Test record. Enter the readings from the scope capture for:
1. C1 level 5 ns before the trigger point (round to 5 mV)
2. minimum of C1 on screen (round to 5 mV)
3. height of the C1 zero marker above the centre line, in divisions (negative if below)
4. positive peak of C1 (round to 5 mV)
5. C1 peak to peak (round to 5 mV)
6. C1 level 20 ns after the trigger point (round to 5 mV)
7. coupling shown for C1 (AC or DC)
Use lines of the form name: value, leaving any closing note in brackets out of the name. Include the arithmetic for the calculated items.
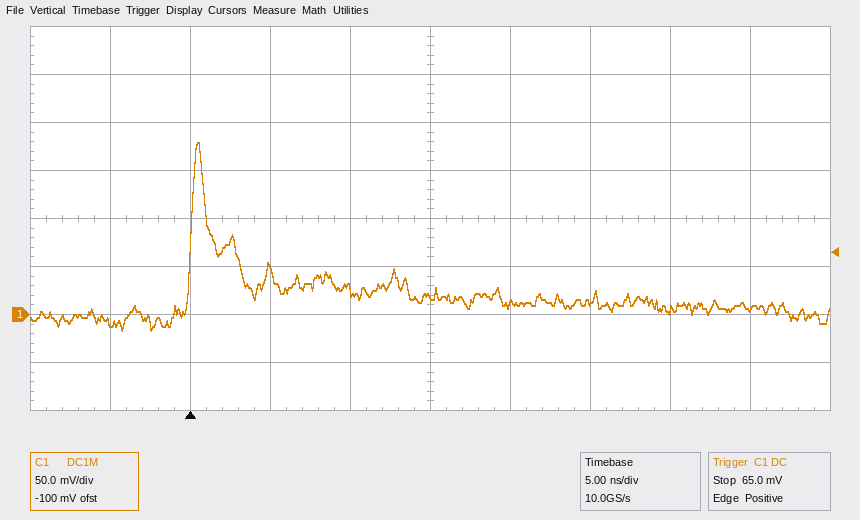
C1 level 5 ns before the trigger point: -10 mV
minimum of C1 on screen: -15 mV
height of the C1 zero marker above the centre line, in divisions: -2.0 div
positive peak of C1: 180 mV
C1 peak to peak: 180 mV − (-15 mV) = 195 mV
C1 level 20 ns after the trigger point: 10 mV
coupling shown for C1: DC
